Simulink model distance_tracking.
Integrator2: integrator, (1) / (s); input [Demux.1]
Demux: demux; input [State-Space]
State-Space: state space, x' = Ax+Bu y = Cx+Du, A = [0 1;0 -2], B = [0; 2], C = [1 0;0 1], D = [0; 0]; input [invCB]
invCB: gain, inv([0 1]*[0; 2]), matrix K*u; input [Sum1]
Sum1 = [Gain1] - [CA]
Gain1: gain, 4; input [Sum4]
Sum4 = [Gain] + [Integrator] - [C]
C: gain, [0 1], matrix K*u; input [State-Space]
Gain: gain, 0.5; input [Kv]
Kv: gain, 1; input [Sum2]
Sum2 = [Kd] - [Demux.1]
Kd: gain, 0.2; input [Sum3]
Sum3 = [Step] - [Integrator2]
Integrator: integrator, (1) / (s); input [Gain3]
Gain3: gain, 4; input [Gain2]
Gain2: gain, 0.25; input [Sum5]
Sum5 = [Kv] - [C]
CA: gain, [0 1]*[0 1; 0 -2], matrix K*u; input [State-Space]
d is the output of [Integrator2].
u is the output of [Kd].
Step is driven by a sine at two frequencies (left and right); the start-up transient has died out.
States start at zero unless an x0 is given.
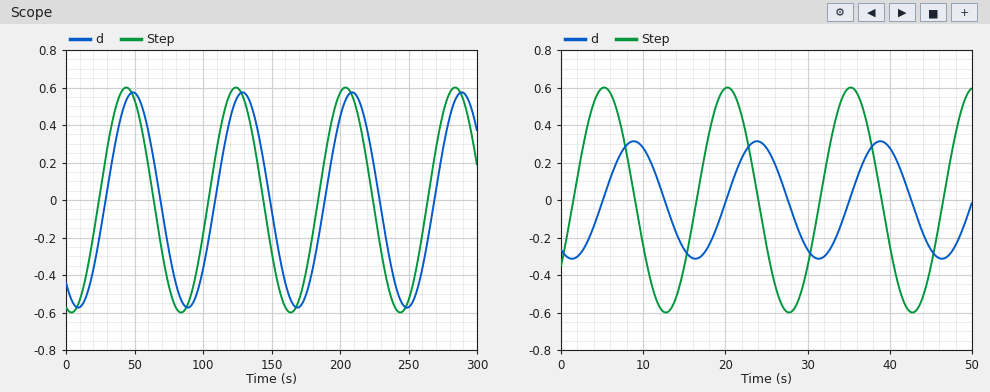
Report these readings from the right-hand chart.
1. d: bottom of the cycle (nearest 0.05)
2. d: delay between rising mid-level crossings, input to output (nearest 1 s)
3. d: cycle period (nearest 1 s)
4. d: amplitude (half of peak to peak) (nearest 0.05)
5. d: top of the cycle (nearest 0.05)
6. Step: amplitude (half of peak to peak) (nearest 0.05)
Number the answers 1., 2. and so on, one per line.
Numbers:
1. -0.30
2. 4 s
3. 15 s
4. 0.30
5. 0.30
6. 0.60
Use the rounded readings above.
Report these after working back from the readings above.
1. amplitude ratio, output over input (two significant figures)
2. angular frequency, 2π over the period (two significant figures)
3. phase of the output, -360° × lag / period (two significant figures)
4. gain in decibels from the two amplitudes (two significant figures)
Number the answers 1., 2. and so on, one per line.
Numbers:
1. 0.50
2. 0.42 rad/s
3. -96°
4. -6.0 dB
